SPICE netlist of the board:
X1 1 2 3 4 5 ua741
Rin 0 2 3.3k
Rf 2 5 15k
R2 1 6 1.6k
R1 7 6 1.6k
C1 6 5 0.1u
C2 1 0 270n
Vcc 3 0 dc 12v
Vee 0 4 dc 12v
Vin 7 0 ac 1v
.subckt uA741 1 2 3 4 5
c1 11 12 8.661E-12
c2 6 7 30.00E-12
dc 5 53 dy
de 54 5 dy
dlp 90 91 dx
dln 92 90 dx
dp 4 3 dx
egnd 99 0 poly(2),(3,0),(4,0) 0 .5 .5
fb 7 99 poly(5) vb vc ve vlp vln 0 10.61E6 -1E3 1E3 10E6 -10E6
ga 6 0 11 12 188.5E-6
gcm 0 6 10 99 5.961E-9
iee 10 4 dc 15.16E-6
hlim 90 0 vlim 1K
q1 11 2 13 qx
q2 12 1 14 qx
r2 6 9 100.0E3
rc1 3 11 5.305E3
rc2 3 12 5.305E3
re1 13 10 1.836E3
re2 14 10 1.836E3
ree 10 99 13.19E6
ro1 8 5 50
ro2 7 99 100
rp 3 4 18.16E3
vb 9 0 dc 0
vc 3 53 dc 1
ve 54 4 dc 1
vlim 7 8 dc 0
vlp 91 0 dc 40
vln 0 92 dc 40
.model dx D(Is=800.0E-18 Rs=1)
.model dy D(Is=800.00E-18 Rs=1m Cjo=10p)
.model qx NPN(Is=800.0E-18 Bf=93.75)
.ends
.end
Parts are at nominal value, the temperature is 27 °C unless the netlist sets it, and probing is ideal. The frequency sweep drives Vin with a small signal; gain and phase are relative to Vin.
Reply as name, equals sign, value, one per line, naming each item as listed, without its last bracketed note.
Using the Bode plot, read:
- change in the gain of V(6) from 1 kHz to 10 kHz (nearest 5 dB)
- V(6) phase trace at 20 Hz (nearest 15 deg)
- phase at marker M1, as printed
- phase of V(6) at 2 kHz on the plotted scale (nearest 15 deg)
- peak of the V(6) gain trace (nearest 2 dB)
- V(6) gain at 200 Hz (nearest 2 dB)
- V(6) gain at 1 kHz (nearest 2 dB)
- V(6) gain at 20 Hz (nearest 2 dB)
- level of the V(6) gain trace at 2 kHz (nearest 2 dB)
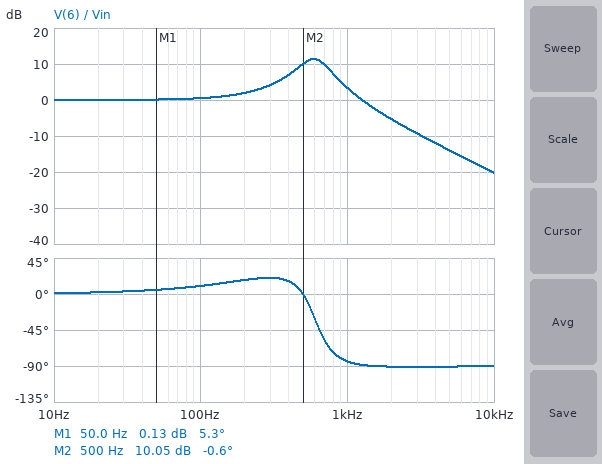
change in the gain of V(6) from 1 kHz to 10 kHz = -25 dB
V(6) phase trace at 20 Hz = 0 deg
phase at marker M1, as printed = 5.3 deg
phase of V(6) at 2 kHz on the plotted scale = -90 deg
peak of the V(6) gain trace = 12 dB
V(6) gain at 200 Hz = 2 dB
V(6) gain at 1 kHz = 4 dB
V(6) gain at 20 Hz = 0 dB
level of the V(6) gain trace at 2 kHz = -6 dB
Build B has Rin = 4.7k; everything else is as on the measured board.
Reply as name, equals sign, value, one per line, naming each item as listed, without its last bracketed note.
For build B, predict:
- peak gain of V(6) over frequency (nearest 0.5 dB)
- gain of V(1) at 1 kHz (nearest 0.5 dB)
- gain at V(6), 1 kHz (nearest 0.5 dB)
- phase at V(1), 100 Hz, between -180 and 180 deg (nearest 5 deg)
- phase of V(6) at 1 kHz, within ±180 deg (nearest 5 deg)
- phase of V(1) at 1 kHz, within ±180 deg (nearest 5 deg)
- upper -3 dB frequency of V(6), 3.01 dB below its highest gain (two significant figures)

peak gain of V(6) over frequency = 3.5 dB
gain of V(1) at 1 kHz = -9.0 dB
gain at V(6), 1 kHz = 0 dB
phase at V(1), 100 Hz, between -180 and 180 deg = -15 deg
phase of V(6) at 1 kHz, within ±180 deg = -60 deg
phase of V(1) at 1 kHz, within ±180 deg = -130 deg
upper -3 dB frequency of V(6), 3.01 dB below its highest gain = 990 Hz
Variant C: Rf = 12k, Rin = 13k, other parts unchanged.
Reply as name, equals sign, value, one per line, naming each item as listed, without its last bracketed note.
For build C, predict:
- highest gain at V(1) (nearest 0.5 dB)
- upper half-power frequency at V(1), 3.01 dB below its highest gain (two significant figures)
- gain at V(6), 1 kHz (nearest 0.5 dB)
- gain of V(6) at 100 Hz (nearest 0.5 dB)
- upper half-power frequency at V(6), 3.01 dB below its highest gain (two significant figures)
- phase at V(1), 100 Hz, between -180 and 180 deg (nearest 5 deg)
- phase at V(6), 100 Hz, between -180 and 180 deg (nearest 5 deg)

highest gain at V(1) = 0 dB
upper half-power frequency at V(1), 3.01 dB below its highest gain = 260 Hz
gain at V(6), 1 kHz = -4.5 dB
gain of V(6) at 100 Hz = -0.5 dB
upper half-power frequency at V(6), 3.01 dB below its highest gain = 600 Hz
phase at V(1), 100 Hz, between -180 and 180 deg = -25 deg
phase at V(6), 100 Hz, between -180 and 180 deg = -10 deg
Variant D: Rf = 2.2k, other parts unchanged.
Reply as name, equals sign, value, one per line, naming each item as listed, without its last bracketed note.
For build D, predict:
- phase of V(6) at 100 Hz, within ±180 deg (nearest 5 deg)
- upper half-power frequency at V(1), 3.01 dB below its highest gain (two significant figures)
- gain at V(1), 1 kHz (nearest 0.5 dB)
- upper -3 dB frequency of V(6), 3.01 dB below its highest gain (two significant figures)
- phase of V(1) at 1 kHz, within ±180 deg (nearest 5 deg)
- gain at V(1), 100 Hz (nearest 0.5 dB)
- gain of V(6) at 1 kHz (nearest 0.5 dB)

phase of V(6) at 100 Hz, within ±180 deg = -10 deg
upper half-power frequency at V(1), 3.01 dB below its highest gain = 240 Hz
gain at V(1), 1 kHz = -14.0 dB
upper -3 dB frequency of V(6), 3.01 dB below its highest gain = 490 Hz
phase of V(1) at 1 kHz, within ±180 deg = -110 deg
gain at V(1), 100 Hz = -0.5 dB
gain of V(6) at 1 kHz = -5.0 dB
